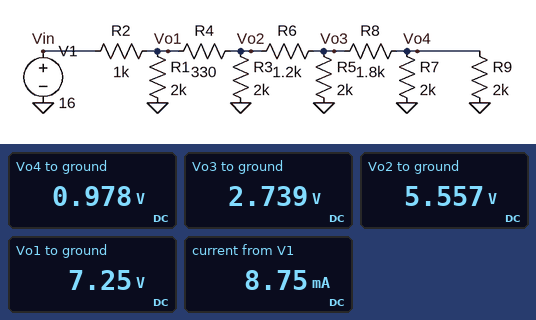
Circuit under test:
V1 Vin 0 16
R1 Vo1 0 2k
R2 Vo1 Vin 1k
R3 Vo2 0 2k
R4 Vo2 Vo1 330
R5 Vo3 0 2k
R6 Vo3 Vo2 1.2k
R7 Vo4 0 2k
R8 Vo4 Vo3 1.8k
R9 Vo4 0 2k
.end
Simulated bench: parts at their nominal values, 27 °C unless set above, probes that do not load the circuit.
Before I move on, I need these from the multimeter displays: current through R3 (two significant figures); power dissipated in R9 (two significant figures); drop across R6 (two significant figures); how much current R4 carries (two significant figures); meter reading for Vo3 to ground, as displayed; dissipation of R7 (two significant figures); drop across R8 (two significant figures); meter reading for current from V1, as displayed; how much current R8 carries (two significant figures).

2.8 mA
480 µW
2.8 V
5.1 mA
2.739 V
480 µW
1.8 V
8.75 mA
980 µA
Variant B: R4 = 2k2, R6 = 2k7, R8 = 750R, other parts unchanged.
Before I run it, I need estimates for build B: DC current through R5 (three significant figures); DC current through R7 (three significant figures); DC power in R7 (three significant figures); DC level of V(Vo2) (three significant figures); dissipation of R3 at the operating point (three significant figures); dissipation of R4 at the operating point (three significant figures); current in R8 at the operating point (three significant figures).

425 µA
243 µA
118 µW
3.31 V
5.48 mW
14.5 mW
486 µA
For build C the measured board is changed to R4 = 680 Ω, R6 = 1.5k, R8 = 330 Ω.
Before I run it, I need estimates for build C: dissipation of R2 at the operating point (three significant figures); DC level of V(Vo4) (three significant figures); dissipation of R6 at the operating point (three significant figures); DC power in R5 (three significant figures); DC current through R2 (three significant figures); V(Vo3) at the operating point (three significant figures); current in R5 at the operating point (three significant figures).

68.5 mW
1.23 V
6.33 mW
1.35 mW
8.28 mA
1.64 V
820 µA
